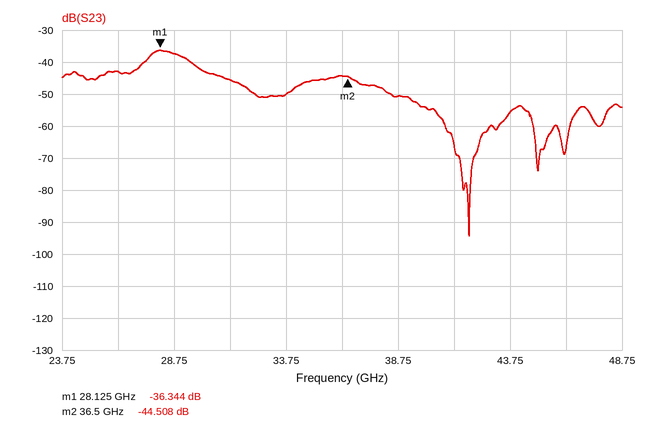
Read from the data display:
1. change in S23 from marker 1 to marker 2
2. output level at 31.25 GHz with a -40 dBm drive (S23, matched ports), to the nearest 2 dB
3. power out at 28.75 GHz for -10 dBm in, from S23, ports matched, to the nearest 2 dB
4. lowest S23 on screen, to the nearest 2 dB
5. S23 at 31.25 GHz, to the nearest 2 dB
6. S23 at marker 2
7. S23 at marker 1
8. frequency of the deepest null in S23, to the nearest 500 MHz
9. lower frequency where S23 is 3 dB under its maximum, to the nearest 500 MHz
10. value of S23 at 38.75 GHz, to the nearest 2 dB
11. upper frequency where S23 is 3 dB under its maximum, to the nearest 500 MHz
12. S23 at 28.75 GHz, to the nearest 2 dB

-8.164 dB
-86 dBm
-48 dBm
-94 dB
-46 dB
-44.508 dB
-36.344 dB
42.0 GHz
27.5 GHz
-50 dB
29.5 GHz
-38 dB
